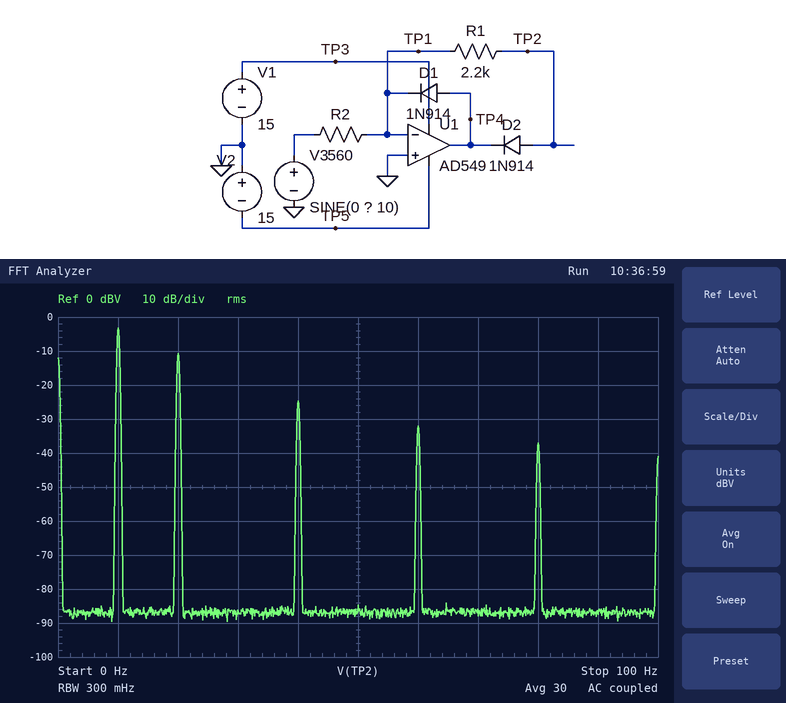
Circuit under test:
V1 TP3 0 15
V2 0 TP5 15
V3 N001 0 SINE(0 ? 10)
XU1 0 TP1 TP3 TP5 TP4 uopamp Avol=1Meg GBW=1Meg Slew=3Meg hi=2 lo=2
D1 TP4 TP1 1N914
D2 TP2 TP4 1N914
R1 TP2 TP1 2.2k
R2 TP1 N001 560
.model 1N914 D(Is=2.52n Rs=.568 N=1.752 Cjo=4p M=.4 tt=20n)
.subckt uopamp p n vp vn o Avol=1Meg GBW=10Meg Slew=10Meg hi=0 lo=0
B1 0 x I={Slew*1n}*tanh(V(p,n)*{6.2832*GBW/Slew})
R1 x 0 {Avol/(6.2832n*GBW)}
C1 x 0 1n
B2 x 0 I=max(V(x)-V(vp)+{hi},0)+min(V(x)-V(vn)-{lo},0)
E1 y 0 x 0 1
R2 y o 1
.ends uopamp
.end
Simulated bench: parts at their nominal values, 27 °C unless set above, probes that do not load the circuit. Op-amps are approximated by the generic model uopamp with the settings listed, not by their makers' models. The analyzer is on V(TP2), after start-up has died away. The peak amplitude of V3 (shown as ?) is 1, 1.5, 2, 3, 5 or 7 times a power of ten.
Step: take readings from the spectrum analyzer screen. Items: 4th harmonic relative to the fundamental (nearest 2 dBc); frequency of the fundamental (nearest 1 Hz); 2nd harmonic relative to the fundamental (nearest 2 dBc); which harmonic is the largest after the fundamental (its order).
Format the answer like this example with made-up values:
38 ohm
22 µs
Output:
-22 dBc
10 Hz
-8 dBc
2
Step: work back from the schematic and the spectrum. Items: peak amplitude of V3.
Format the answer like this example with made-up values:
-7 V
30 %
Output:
500 mV
